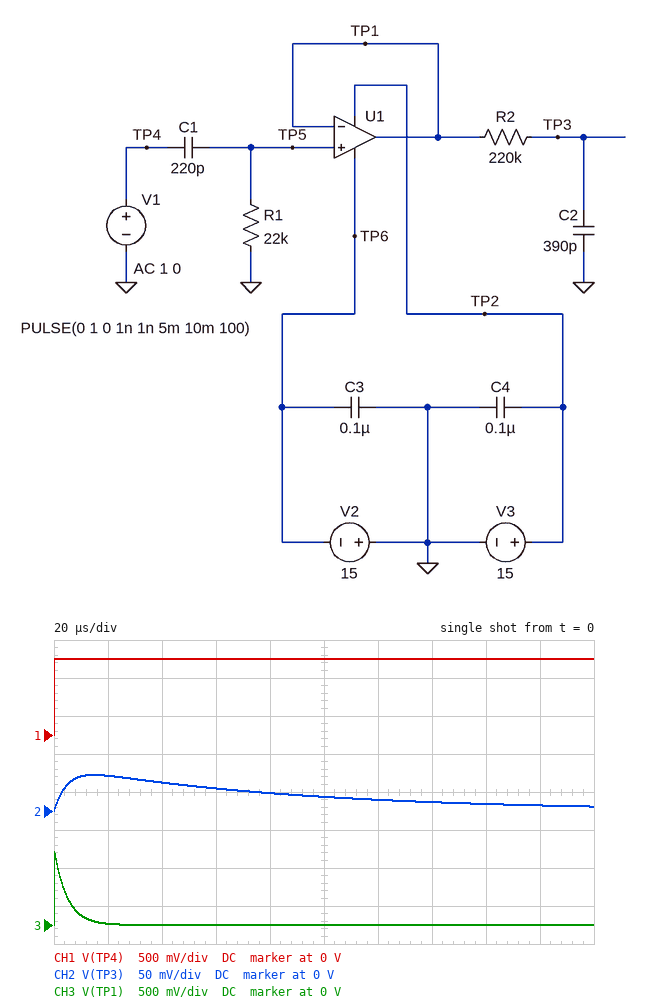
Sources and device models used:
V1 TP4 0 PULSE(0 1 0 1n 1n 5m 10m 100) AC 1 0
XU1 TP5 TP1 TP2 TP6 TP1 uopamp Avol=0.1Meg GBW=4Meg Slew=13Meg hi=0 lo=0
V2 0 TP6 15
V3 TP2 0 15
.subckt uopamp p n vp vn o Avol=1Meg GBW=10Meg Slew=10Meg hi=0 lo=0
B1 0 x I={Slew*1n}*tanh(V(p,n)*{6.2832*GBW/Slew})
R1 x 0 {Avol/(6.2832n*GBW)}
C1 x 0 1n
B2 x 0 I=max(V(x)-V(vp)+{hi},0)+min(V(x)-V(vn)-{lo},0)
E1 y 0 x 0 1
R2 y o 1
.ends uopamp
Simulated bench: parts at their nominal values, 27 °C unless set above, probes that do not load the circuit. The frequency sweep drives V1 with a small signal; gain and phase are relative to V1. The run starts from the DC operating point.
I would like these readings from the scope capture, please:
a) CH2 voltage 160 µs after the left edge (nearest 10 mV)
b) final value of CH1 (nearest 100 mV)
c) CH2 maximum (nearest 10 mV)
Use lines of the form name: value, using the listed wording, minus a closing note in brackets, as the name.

CH2 voltage 160 µs after the left edge: 10 mV
final value of CH1: 1.0 V
CH2 maximum: 50 mV
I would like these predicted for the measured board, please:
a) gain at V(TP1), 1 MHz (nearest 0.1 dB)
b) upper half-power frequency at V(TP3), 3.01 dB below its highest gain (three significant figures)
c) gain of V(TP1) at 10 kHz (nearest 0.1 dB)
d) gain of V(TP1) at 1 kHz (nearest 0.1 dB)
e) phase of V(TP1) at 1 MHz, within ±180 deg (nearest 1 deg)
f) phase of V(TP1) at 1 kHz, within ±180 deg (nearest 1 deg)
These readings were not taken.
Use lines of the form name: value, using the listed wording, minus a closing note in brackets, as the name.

gain at V(TP1), 1 MHz: -0.3 dB
upper half-power frequency at V(TP3), 3.01 dB below its highest gain: 36.4 kHz
gain of V(TP1) at 10 kHz: -10.7 dB
gain of V(TP1) at 1 kHz: -30.3 dB
phase of V(TP1) at 1 MHz, within ±180 deg: -12 deg
phase of V(TP1) at 1 kHz, within ±180 deg: 88 deg
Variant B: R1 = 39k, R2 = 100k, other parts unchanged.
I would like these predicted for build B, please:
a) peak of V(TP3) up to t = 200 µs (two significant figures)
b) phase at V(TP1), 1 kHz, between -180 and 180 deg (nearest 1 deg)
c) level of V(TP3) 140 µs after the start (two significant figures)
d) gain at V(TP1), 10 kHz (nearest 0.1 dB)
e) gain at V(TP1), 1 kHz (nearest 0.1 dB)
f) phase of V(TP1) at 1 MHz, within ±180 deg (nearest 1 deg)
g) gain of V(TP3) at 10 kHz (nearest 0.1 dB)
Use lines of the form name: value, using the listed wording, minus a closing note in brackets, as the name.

peak of V(TP3) up to t = 200 µs: 140 mV
phase at V(TP1), 1 kHz, between -180 and 180 deg: 87 deg
level of V(TP3) 140 µs after the start: 7.8 mV
gain at V(TP1), 10 kHz: -6.5 dB
gain at V(TP1), 1 kHz: -25.4 dB
phase of V(TP1) at 1 MHz, within ±180 deg: -13 deg
gain of V(TP3) at 10 kHz: -14.9 dB
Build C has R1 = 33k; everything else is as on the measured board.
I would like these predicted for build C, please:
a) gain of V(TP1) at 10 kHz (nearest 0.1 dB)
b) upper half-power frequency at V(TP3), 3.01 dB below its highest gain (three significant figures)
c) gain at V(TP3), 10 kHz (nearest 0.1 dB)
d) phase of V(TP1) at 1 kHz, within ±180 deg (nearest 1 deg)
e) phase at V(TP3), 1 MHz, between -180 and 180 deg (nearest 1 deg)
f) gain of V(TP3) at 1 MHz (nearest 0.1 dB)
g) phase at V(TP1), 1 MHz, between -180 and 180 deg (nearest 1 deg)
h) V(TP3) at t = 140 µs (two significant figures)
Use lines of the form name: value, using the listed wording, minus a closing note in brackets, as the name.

gain of V(TP1) at 10 kHz: -7.6 dB
upper half-power frequency at V(TP3), 3.01 dB below its highest gain: 25.4 kHz
gain at V(TP3), 10 kHz: -22.4 dB
phase of V(TP1) at 1 kHz, within ±180 deg: 87 deg
phase at V(TP3), 1 MHz, between -180 and 180 deg: -103 deg
gain of V(TP3) at 1 MHz: -54.9 dB
phase at V(TP1), 1 MHz, between -180 and 180 deg: -13 deg
V(TP3) at t = 140 µs: 18 mV
